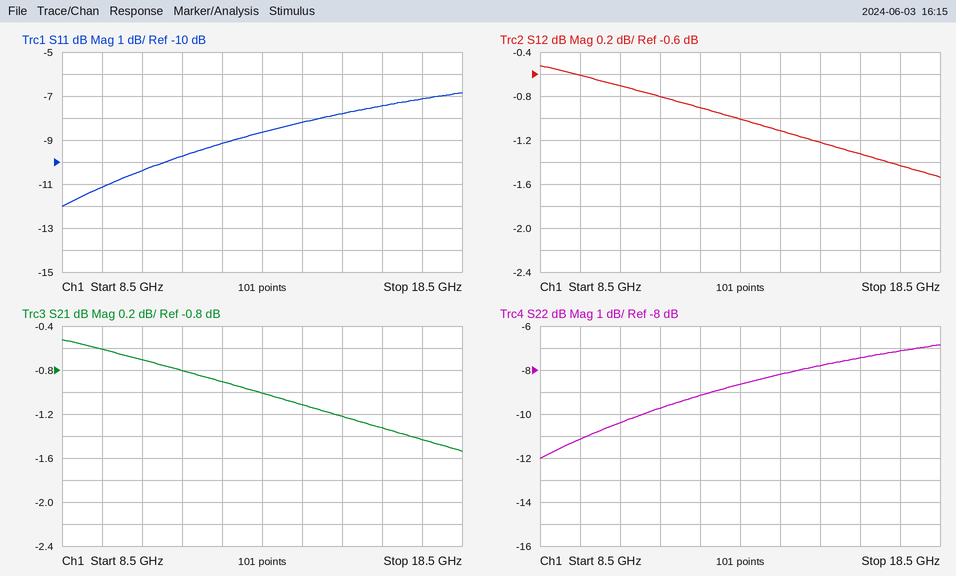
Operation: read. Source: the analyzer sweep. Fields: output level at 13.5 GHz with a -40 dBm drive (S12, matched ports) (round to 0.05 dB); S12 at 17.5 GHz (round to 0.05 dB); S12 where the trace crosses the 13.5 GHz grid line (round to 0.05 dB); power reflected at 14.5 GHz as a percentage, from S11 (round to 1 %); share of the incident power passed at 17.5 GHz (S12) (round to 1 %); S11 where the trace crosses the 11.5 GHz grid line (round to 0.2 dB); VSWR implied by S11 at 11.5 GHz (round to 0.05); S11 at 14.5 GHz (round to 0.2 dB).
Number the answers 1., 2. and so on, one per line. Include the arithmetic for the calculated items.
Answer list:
1. -40 dBm + (-1.00 dB) = -41.00 dBm
2. -1.45 dB
3. -1.00 dB
4. 10^(-8.2/10) ≈ 15 %
5. 10^(-1.45/10) ≈ 72 %
6. -9.8 dB
7. |Γ| = 10^(-9.8/20) = 0.3236; VSWR = (1 + 0.3236)/(1 − 0.3236) ≈ 1.96, so 1.95 to the nearest 0.05
8. -8.2 dB
